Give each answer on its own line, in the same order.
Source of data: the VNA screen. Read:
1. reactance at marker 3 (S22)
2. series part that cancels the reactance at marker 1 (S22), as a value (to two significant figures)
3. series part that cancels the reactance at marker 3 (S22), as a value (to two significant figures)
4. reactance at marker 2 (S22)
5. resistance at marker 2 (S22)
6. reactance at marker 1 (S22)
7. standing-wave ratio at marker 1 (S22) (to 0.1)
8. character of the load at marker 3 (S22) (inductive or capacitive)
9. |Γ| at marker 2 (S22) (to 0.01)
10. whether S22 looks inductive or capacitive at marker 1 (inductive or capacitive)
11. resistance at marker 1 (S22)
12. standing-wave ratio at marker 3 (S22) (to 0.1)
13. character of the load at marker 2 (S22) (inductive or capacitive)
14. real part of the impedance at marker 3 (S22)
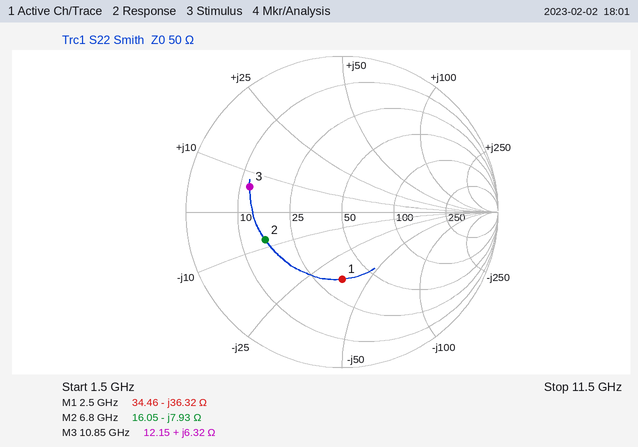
+6.32 Ω
2.3 nH
2.3 pF
-7.93 Ω
16.05 Ω
-36.32 Ω
2.5
inductive
0.52
capacitive
34.46 Ω
4.2
capacitive
12.15 Ω
